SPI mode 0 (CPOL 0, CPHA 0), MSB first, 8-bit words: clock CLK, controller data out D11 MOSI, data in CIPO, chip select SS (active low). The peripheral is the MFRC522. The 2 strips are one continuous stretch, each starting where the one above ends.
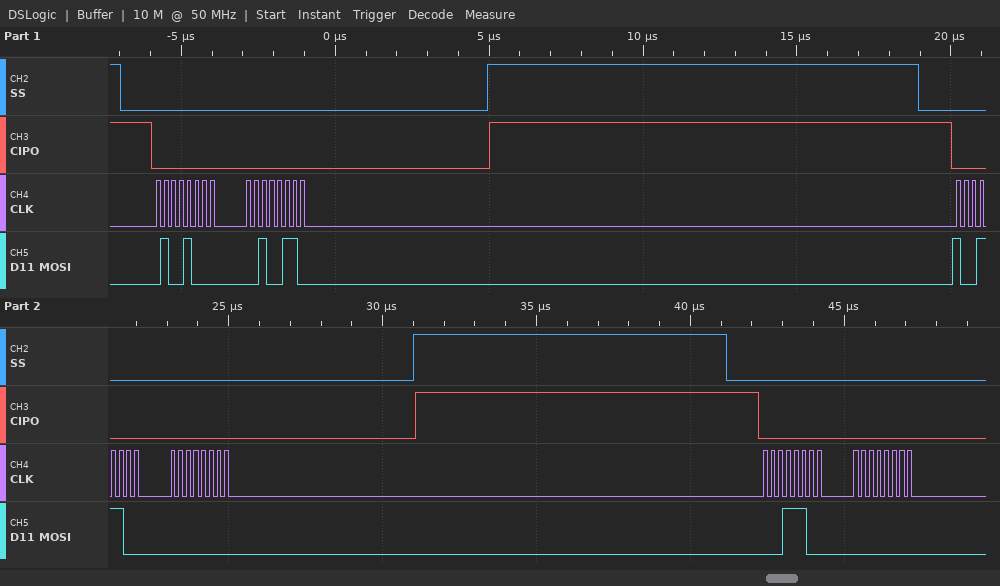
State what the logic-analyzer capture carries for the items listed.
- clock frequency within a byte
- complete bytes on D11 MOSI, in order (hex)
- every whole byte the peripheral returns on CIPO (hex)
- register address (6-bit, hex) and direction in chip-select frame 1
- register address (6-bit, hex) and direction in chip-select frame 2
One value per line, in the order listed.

4 MHz
48 26 9C 00 1C 00
00 00 00 00 00 00
0x24 write
0x0E read
